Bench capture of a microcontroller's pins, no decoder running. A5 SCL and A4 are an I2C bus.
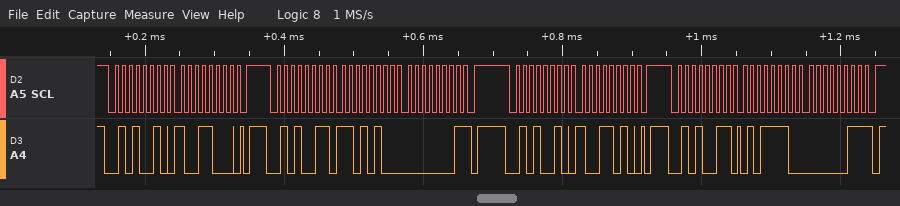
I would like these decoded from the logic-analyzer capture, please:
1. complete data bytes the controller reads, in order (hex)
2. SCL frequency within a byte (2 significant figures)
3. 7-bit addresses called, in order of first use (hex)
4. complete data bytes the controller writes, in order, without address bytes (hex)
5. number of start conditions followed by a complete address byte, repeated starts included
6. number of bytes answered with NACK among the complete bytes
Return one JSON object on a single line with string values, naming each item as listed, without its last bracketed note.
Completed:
{"complete data bytes the controller reads, in order": "D4 01 5E 03", "SCL frequency within a byte": "100 kHz", "7-bit addresses called, in order of first use": "0x29", "complete data bytes the controller writes, in order, without address bytes": "98 9A", "number of start conditions followed by a complete address byte, repeated starts included": "4", "number of bytes answered with NACK among the complete bytes": "2"}
